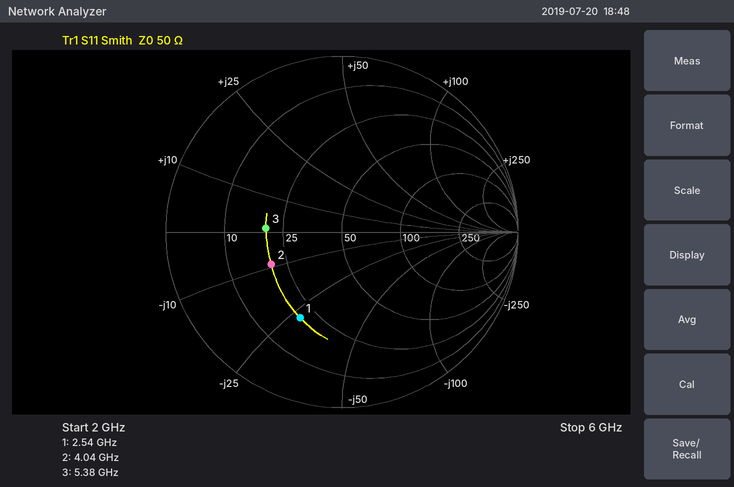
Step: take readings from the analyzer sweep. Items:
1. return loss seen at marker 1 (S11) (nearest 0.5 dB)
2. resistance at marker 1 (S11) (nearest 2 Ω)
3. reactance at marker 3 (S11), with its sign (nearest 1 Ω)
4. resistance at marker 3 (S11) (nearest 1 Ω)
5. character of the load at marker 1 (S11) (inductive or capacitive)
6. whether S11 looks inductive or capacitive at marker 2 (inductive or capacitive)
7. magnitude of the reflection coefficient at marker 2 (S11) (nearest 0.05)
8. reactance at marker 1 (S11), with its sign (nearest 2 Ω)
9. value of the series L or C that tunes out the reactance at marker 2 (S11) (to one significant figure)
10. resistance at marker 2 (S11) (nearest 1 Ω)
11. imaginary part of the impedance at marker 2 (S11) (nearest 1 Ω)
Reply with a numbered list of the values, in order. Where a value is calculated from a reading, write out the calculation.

1. 5.5 dB
2. 20 Ω
3. +1 Ω
4. 20 Ω
5. capacitive
6. capacitive
7. 0.45
8. -28 Ω
9. L = 9 Ω/(2π × 4.04 GHz) ≈ 355 pH, so 400 pH to one significant figure
10. 20 Ω
11. -9 Ω
